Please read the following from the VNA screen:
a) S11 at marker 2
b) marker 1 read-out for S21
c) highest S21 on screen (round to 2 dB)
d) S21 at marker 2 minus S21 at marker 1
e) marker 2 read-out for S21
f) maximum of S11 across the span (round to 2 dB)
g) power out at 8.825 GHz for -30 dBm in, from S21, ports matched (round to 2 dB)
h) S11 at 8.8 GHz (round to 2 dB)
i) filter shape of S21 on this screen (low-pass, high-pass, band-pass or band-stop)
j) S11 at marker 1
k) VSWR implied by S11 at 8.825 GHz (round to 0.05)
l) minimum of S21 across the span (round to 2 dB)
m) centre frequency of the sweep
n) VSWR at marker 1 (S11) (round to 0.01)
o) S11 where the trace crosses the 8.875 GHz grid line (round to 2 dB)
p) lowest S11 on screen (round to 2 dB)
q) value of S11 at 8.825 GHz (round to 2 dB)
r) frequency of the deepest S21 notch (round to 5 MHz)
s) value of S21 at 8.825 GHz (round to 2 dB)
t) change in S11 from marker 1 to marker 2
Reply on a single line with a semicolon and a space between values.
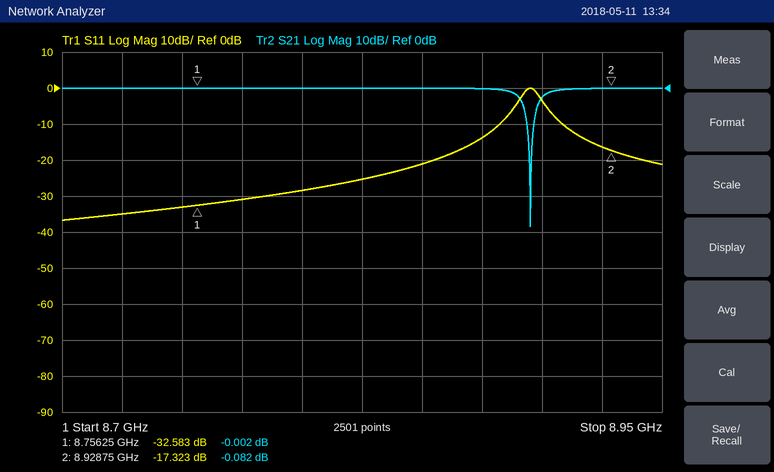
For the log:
-17.323 dB; -0.002 dB; 0 dB; -0.080 dB; -0.082 dB; 0 dB; -30 dBm; -28 dB; band-stop; -32.583 dB; 1.10; -38 dB; 8.825 GHz; 1.05; -14 dB; -36 dB; -26 dB; 8.895 GHz; 0 dB; 15.260 dB
